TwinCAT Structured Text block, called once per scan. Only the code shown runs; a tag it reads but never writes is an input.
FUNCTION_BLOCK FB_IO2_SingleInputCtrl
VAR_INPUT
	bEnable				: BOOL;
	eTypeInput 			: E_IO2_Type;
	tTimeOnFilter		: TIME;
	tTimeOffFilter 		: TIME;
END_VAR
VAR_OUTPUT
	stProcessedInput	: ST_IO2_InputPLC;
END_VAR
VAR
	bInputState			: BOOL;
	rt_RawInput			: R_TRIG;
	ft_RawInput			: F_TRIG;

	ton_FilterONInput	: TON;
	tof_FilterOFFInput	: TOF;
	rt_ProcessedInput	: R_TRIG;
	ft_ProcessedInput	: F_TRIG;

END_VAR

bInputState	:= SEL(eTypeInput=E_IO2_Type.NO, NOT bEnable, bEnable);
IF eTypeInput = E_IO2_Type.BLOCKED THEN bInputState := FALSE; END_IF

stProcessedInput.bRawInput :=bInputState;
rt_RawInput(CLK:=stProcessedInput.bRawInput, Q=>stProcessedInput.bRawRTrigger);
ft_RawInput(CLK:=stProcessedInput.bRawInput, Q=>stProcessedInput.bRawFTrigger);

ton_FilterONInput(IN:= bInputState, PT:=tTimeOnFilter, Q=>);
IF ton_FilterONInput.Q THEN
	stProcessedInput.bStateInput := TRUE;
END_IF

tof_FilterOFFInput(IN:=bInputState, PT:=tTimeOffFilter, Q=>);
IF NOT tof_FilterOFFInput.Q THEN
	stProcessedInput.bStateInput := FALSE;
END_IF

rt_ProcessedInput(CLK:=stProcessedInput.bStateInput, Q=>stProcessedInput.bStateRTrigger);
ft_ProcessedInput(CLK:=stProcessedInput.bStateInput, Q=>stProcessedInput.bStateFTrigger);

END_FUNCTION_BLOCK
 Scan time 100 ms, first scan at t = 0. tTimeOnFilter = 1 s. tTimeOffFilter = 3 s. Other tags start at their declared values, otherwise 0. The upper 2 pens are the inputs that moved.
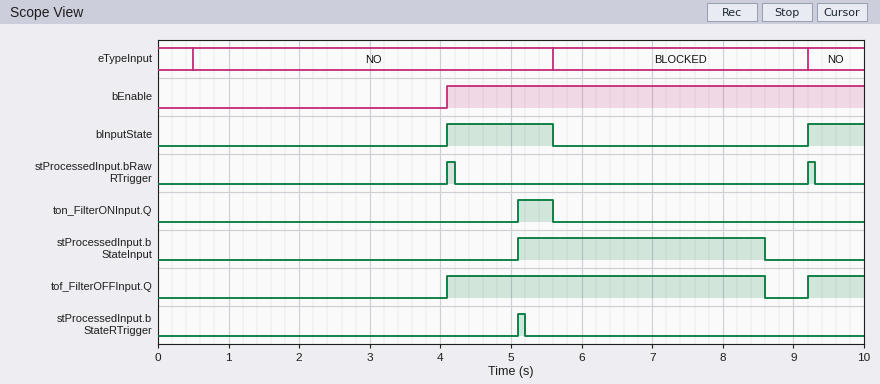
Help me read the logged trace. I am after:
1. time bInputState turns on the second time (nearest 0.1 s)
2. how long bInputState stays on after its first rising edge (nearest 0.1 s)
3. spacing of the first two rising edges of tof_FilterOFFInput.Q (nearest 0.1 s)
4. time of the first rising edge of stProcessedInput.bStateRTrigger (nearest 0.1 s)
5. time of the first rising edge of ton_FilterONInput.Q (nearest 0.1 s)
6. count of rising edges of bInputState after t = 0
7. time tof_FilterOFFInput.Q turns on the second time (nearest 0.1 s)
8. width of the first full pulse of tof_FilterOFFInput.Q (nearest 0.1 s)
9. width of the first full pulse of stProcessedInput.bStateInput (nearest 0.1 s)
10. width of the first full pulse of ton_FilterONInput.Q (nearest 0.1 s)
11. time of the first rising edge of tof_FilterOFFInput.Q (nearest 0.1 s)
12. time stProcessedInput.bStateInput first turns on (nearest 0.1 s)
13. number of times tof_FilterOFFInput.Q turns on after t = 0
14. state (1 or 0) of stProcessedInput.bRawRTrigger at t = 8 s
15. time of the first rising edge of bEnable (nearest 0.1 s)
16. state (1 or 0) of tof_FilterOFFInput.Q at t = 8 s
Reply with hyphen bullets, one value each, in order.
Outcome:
- 9.2 s
- 1.5 s
- 5.1 s
- 5.1 s
- 5.1 s
- 2
- 9.2 s
- 4.5 s
- 3.5 s
- 0.5 s
- 4.1 s
- 5.1 s
- 2
- 0
- 4.1 s
- 1
